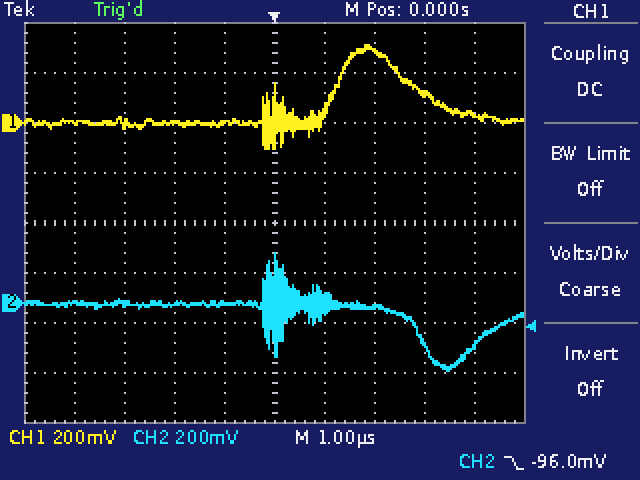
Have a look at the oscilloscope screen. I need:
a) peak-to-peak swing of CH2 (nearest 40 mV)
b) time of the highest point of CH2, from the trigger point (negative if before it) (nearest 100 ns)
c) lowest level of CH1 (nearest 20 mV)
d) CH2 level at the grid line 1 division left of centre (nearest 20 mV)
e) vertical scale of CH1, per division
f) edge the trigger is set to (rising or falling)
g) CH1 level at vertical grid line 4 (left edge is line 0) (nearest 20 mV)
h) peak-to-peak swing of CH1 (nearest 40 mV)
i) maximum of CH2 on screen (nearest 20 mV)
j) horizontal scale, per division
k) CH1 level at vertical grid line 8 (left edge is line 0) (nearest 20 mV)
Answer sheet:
480 mV
0.0 µs
-100 mV
0 mV
200 mV
falling
0 mV
400 mV
200 mV
1 µs
120 mV
